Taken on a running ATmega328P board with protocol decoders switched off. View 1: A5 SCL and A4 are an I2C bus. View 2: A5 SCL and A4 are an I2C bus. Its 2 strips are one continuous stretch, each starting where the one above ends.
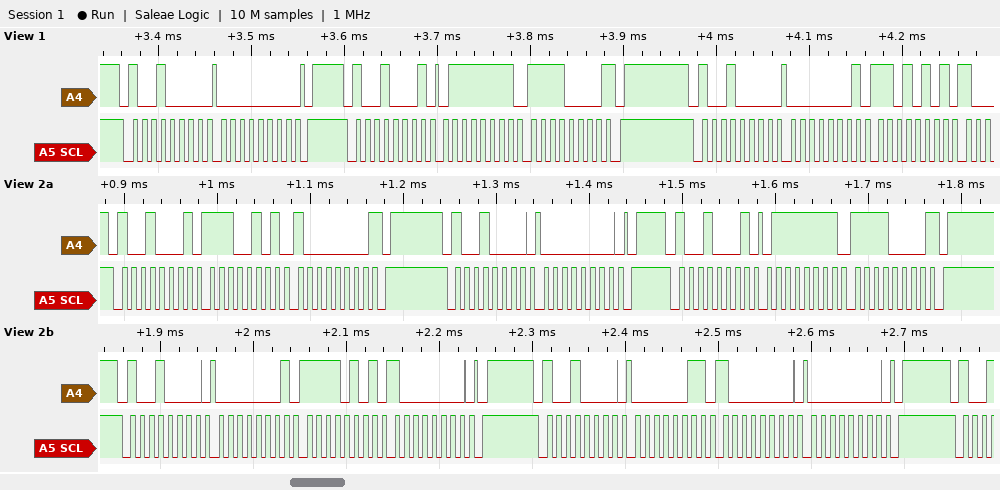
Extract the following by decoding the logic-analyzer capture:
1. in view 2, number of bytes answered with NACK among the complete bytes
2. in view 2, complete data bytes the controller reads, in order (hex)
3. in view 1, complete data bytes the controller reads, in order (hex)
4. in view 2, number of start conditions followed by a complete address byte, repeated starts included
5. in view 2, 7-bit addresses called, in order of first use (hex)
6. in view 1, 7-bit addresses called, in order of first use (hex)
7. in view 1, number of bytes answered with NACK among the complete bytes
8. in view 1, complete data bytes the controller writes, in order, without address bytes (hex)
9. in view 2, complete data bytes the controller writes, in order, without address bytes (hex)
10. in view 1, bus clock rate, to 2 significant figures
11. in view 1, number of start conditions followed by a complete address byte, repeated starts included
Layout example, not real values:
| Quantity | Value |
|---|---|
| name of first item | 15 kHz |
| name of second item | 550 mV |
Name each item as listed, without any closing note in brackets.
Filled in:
| Quantity | Value |
|---|---|
| in view 2, number of bytes answered with NACK among the complete bytes | 2 |
| in view 2, complete data bytes the controller reads, in order | E5 80 7F F0 |
| in view 1, complete data bytes the controller reads, in order | 7F F0 |
| in view 2, number of start conditions followed by a complete address byte, repeated starts included | 5 |
| in view 2, 7-bit addresses called, in order of first use | 0x48 |
| in view 1, 7-bit addresses called, in order of first use | 0x48 |
| in view 1, number of bytes answered with NACK among the complete bytes | 1 |
| in view 1, complete data bytes the controller writes, in order, without address bytes | 00 01 D5 |
| in view 2, complete data bytes the controller writes, in order, without address bytes | 00 01 F5 80 03 80 00 |
| in view 1, bus clock rate, to 2 significant figures | 100 kHz |
| in view 1, number of start conditions followed by a complete address byte, repeated starts included | 3 |
